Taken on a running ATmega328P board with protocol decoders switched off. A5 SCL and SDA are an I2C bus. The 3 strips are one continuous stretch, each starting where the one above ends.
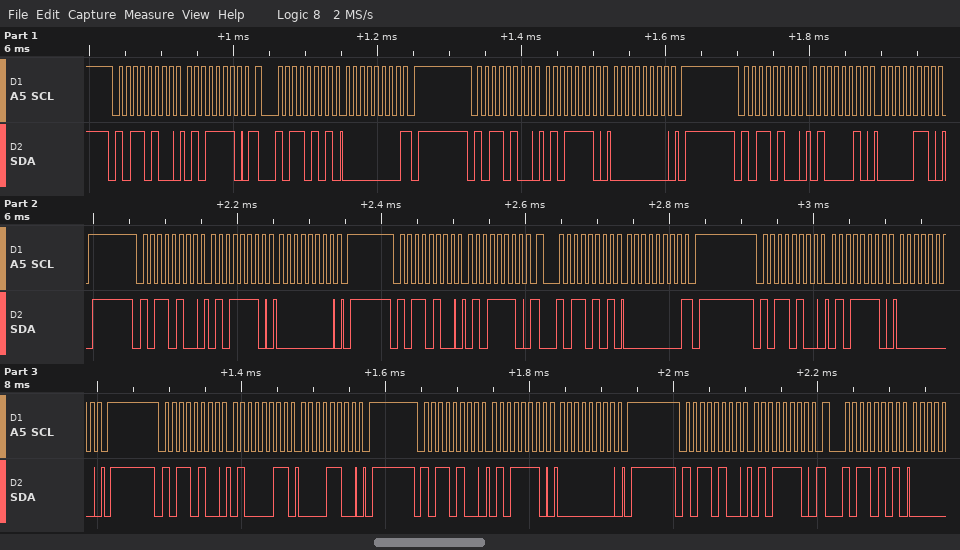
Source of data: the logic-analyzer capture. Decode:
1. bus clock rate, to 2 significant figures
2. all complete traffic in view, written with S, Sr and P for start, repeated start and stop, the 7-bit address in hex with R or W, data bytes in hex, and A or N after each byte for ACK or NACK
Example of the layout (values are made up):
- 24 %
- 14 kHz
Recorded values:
- 100 kHz
- S 5AW A 5E A Sr 5AR A 00 N P S 5AW A 5E A 00 A P S 5AW A 42 A 06 A P S 5AW A 5E A 00 A P S 5AW A 5E A Sr 5AR A 00 N P S 5AW A 5E A 00 A P S 5AW A 43 A 0C A P S 5AW A 5E A 00 A P S 5AW A 5E A Sr 5AR A
